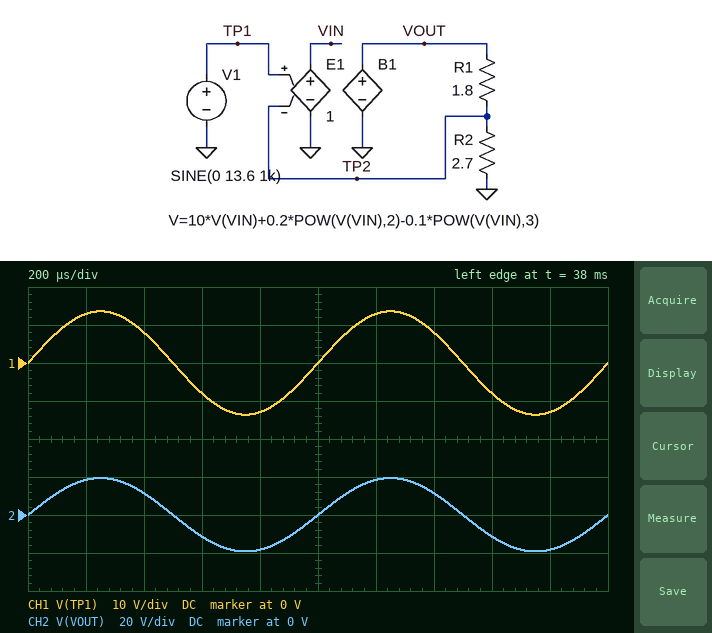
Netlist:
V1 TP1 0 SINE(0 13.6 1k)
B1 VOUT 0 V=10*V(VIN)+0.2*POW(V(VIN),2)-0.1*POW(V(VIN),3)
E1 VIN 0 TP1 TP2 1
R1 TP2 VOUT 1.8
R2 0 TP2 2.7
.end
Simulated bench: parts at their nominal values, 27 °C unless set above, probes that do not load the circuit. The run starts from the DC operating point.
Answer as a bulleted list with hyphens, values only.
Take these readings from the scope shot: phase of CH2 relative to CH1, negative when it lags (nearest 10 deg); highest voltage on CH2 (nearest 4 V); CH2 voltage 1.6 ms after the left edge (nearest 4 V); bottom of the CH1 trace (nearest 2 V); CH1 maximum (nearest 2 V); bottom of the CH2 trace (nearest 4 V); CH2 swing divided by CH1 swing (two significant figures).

- 0 deg
- 20 V
- -12 V
- -14 V
- 14 V
- -20 V
- 1.4
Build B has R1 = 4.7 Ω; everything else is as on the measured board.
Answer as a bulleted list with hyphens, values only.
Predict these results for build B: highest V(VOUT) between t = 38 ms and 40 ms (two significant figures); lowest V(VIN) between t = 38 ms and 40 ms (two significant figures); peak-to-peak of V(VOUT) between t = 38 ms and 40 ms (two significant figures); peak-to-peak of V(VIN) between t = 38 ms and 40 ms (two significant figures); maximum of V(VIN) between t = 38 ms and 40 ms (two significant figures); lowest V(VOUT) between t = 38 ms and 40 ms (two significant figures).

- 29 V
- -3.4 V
- 57 V
- 6.4 V
- 3.0 V
- -28 V
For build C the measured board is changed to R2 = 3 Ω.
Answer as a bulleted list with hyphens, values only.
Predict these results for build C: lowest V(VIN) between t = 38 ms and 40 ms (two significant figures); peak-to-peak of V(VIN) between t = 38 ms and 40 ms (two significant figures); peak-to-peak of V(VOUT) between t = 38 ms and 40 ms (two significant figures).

- -2.0 V
- 3.9 V
- 37 V
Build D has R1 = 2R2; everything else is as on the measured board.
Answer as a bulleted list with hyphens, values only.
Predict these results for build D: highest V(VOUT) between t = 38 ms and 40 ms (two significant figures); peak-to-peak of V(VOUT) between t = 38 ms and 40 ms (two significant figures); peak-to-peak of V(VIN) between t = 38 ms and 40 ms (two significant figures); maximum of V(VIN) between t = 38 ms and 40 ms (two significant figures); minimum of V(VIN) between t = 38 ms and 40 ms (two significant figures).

- 21 V
- 41 V
- 4.4 V
- 2.1 V
- -2.3 V
